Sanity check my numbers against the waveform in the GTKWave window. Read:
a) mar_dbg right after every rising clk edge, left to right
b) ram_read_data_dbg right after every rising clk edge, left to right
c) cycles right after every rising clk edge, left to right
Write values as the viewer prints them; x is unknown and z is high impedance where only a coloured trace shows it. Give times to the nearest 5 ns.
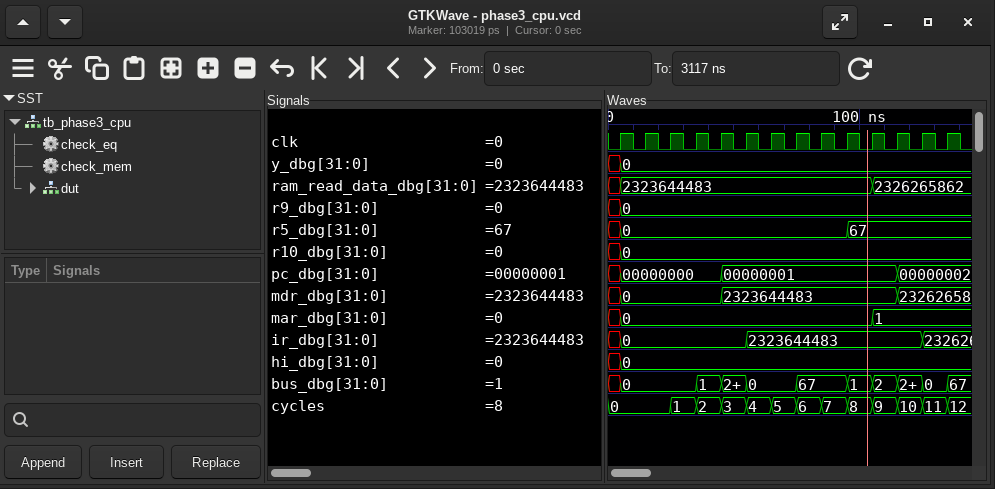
0, 0, 0, 0, 0, 0, 0, 0, 0, 0, 1, 1, 1, 1
2323644483, 2323644483, 2323644483, 2323644483, 2323644483, 2323644483, 2323644483, 2323644483, 2323644483, 2323644483, 2326265862, 2326265862, 2326265862, 2326265862
0, 0, 1, 2, 3, 4, 5, 6, 7, 8, 9, 10, 11, 12
